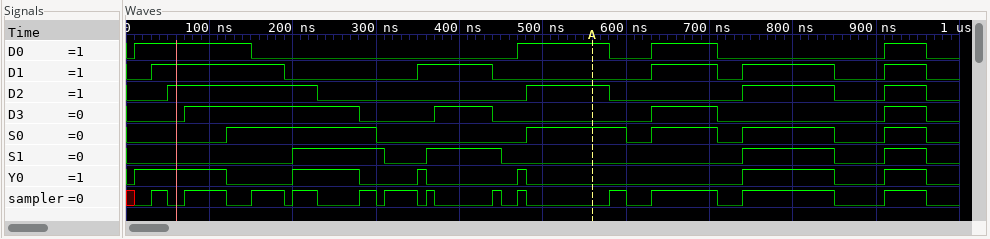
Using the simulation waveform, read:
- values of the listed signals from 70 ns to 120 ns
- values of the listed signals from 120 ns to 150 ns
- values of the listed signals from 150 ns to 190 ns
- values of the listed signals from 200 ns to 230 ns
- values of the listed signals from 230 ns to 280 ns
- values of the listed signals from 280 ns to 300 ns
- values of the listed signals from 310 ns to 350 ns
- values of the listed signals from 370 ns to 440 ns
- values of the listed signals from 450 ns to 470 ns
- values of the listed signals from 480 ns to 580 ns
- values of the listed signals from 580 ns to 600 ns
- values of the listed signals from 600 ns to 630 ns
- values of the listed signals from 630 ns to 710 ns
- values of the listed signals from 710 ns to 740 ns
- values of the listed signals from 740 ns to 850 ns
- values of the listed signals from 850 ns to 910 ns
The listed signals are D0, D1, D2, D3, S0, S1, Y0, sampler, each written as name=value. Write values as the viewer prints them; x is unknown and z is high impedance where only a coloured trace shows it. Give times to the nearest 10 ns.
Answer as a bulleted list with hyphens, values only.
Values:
- D0=1, D1=1, D2=1, D3=1, S0=0, S1=0, Y0=1, sampler=1
- D0=1, D1=1, D2=1, D3=1, S0=1, S1=0, Y0=0, sampler=0
- D0=0, D1=1, D2=1, D3=1, S0=1, S1=0, Y0=0, sampler=1
- D0=0, D1=0, D2=1, D3=1, S0=1, S1=1, Y0=1, sampler=1
- D0=0, D1=0, D2=0, D3=1, S0=1, S1=1, Y0=1, sampler=0
- D0=0, D1=0, D2=0, D3=0, S0=1, S1=1, Y0=0, sampler=1
- D0=0, D1=0, D2=0, D3=0, S0=0, S1=0, Y0=0, sampler=1
- D0=0, D1=1, D2=0, D3=1, S0=0, S1=1, Y0=0, sampler=0
- D0=0, D1=0, D2=0, D3=0, S0=0, S1=0, Y0=0, sampler=0
- D0=1, D1=0, D2=1, D3=0, S0=1, S1=0, Y0=0, sampler=0
- D0=0, D1=0, D2=0, D3=0, S0=1, S1=0, Y0=0, sampler=1
- D0=0, D1=0, D2=0, D3=0, S0=0, S1=0, Y0=0, sampler=0
- D0=1, D1=1, D2=0, D3=1, S0=1, S1=0, Y0=0, sampler=1
- D0=0, D1=0, D2=0, D3=0, S0=0, S1=0, Y0=0, sampler=0
- D0=0, D1=1, D2=1, D3=0, S0=1, S1=1, Y0=1, sampler=1
- D0=0, D1=0, D2=0, D3=0, S0=0, S1=0, Y0=0, sampler=0
